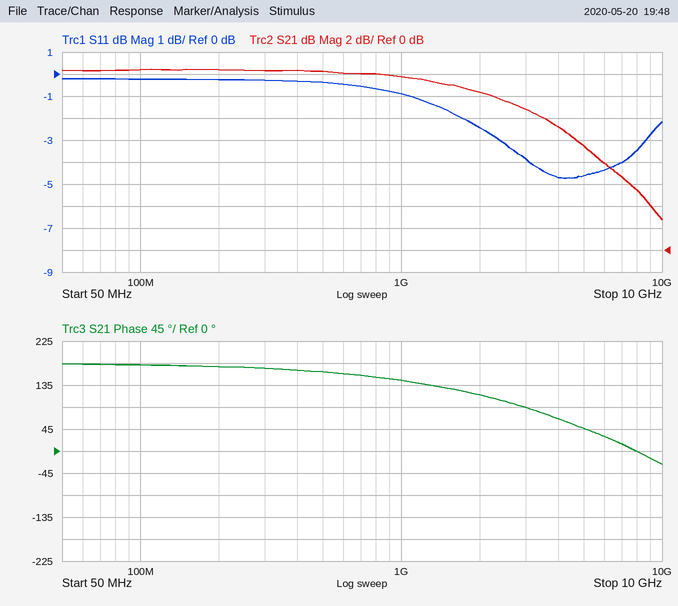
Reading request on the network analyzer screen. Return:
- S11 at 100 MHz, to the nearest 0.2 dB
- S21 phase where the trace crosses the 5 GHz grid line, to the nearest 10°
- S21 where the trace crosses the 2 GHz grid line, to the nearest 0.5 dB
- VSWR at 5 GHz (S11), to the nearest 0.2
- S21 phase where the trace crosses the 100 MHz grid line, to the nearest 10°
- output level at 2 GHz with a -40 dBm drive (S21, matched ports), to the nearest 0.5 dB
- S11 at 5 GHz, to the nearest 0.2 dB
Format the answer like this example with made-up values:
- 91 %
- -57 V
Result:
- -0.2 dB
- 50°
- 14.5 dB
- 3.8
- 180°
- -25.5 dBm
- -4.6 dB
